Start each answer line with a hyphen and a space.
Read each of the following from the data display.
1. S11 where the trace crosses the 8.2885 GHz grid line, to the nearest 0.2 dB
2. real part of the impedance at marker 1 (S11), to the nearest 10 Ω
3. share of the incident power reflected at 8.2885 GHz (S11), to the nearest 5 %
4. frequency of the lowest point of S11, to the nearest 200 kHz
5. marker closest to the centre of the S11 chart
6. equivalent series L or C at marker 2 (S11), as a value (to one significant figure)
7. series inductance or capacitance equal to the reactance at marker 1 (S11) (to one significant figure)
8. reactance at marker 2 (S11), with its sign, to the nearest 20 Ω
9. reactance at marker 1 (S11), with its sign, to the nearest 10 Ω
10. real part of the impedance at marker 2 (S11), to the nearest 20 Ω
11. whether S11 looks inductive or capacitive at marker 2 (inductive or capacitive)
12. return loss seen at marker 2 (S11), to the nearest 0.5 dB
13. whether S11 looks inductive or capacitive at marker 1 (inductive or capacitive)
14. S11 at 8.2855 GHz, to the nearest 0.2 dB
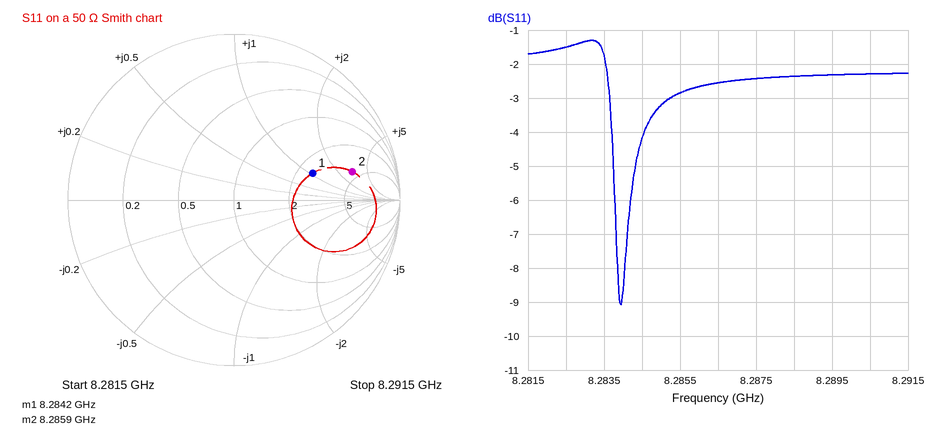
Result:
- -2.4 dB
- 120 Ω
- 60 %
- 8.2840 GHz
- marker 1
- 3 nH
- 1 nH
- +160 Ω
- +50 Ω
- 200 Ω
- inductive
- 2.5 dB
- inductive
- -2.8 dB
